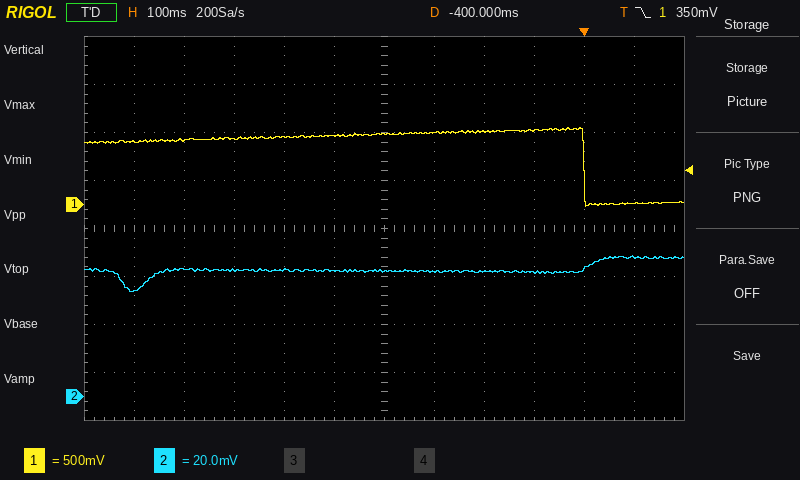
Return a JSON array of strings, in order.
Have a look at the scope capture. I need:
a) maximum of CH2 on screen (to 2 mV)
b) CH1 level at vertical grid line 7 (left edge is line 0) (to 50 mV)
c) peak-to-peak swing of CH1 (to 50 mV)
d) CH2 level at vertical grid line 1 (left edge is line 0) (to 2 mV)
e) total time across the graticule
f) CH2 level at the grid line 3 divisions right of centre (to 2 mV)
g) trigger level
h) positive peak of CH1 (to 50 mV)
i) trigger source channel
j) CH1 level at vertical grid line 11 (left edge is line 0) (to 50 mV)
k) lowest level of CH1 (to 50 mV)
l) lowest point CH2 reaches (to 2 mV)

["58 mV", "750 mV", "800 mV", "44 mV", "1.2 s", "52 mV", "350 mV", "800 mV", "CH1", "0 mV", "0 mV", "44 mV"]
